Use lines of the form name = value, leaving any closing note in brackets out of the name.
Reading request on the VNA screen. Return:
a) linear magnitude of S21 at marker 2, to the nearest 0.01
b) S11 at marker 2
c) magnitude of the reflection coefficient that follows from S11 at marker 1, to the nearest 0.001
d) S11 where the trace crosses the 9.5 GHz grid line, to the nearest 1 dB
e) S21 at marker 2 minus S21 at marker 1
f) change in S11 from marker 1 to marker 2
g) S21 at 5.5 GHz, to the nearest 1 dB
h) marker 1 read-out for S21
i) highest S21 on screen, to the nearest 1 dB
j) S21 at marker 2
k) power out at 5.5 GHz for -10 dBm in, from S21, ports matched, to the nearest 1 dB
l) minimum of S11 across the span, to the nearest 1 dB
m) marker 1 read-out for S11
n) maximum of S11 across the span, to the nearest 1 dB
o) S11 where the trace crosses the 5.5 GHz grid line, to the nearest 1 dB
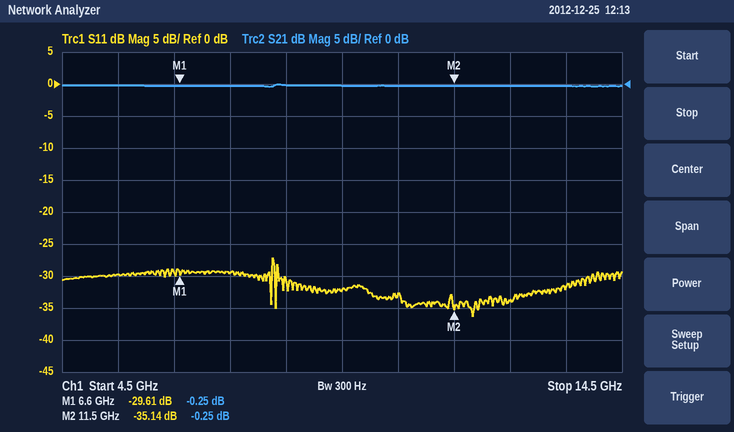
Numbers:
linear magnitude of S21 at marker 2, to the nearest 0.01 = 0.97
S11 at marker 2 = -35.14 dB
magnitude of the reflection coefficient that follows from S11 at marker 1, to the nearest 0.001 = 0.033
S11 where the trace crosses the 9.5 GHz grid line, to the nearest 1 dB = -32 dB
S21 at marker 2 minus S21 at marker 1 = 0.00 dB
change in S11 from marker 1 to marker 2 = -5.53 dB
S21 at 5.5 GHz, to the nearest 1 dB = 0 dB
marker 1 read-out for S21 = -0.25 dB
highest S21 on screen, to the nearest 1 dB = 0 dB
S21 at marker 2 = -0.25 dB
power out at 5.5 GHz for -10 dBm in, from S21, ports matched, to the nearest 1 dB = -10 dBm
minimum of S11 across the span, to the nearest 1 dB = -36 dB
marker 1 read-out for S11 = -29.61 dB
maximum of S11 across the span, to the nearest 1 dB = -27 dB
S11 where the trace crosses the 5.5 GHz grid line, to the nearest 1 dB = -30 dB
